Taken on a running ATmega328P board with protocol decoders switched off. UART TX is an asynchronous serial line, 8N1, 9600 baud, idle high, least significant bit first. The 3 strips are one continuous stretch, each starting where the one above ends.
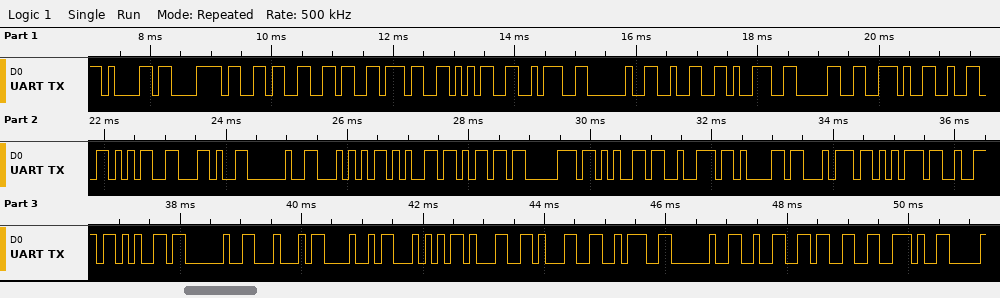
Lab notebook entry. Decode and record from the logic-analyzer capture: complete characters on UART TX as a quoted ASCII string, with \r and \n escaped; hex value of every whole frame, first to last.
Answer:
"ax6675: 290.25, Temperature DHT11: 23."
61 78 36 36 37 35 3A 20 32 39 30 2E 32 35 2C 20 54 65 6D 70 65 72 61 74 75 72 65 20 44 48 54 31 31 3A 20 32 33 2E
